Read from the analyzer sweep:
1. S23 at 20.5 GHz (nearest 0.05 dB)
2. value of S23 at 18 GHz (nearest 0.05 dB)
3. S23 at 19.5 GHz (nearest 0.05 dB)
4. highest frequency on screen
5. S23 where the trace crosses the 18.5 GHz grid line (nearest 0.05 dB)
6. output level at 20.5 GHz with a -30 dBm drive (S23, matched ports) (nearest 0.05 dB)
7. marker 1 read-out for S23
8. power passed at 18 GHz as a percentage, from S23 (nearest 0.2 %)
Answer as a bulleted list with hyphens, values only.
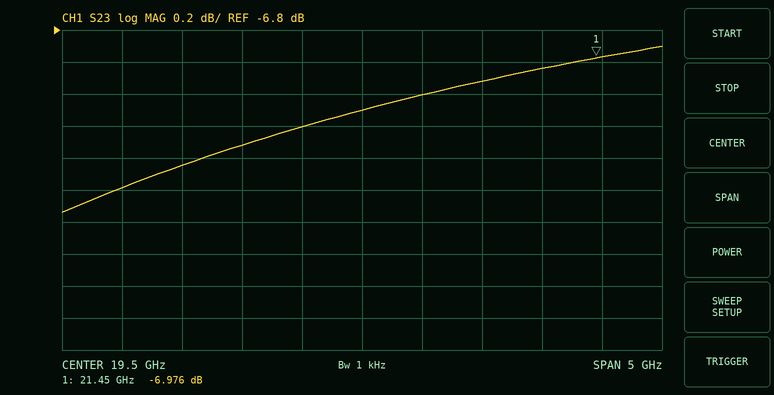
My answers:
- -7.10 dB
- -7.65 dB
- -7.30 dB
- 22 GHz
- -7.50 dB
- -37.10 dBm
- -6.976 dB
- 17.2 %
